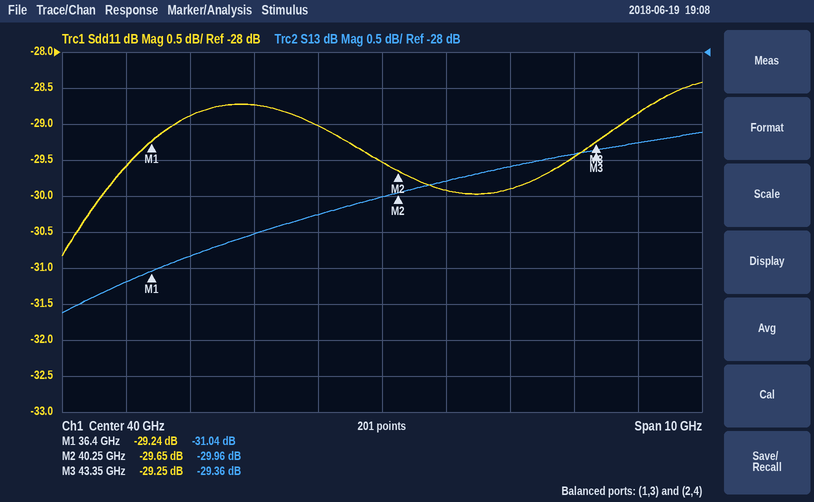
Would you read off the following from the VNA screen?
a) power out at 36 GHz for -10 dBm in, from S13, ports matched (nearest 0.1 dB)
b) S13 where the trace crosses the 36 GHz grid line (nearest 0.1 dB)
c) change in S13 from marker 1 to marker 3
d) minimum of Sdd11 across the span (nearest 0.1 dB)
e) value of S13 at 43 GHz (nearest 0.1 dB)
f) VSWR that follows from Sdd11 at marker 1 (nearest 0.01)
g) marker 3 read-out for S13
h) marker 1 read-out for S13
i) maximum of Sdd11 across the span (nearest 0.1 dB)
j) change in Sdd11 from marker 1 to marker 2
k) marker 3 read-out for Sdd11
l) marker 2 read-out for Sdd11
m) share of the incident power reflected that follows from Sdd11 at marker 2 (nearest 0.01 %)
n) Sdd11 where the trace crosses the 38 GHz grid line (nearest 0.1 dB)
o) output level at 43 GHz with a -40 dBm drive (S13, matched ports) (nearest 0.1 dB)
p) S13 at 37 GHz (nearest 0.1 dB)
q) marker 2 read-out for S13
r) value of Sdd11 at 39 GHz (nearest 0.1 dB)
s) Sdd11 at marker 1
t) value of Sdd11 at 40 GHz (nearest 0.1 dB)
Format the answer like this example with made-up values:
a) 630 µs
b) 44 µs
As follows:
a) -41.2 dBm
b) -31.2 dB
c) 1.68 dB
d) -30.8 dB
e) -29.4 dB
f) 1.07
g) -29.36 dB
h) -31.04 dB
i) -28.4 dB
j) -0.41 dB
k) -29.25 dB
l) -29.65 dB
m) 0.11 %
n) -28.7 dB
o) -69.4 dBm
p) -30.8 dB
q) -29.96 dB
r) -29.0 dB
s) -29.24 dB
t) -29.5 dB
